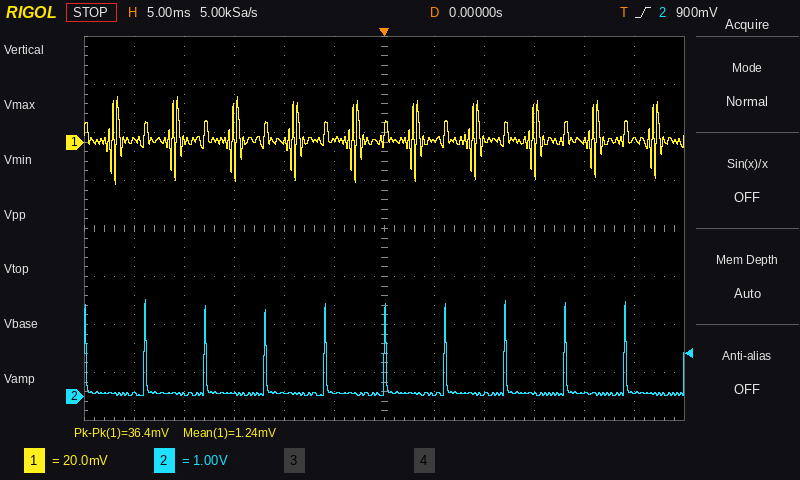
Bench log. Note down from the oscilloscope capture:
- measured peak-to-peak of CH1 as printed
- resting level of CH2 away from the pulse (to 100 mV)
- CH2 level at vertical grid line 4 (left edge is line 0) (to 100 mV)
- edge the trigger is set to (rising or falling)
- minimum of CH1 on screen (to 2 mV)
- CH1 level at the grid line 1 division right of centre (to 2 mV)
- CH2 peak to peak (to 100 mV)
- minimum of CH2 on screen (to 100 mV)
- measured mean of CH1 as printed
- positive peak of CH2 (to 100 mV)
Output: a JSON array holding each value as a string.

["36.4 mV", "100 mV", "100 mV", "rising", "-18 mV", "0 mV", "2.0 V", "0.0 V", "1.24 mV", "2.0 V"]
